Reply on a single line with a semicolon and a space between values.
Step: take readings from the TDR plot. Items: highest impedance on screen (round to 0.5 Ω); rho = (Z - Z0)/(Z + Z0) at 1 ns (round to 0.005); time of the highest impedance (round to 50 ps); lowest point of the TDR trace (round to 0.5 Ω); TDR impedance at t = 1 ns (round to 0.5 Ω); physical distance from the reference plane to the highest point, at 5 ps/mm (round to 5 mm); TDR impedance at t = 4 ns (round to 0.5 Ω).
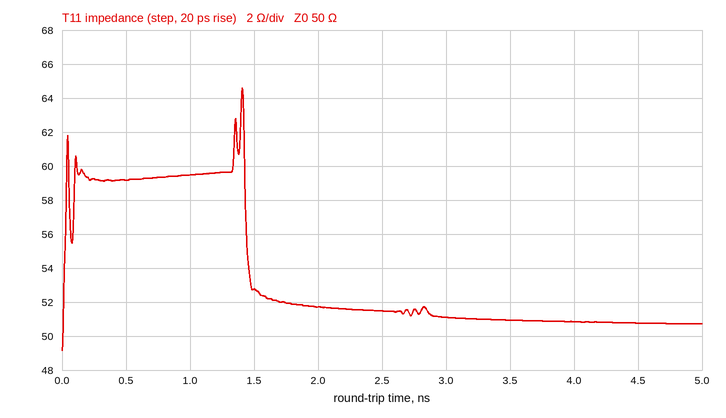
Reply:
64.5 Ω; +0.085; 1.40 ns; 49.0 Ω; 59.5 Ω; 140 mm; 51.0 Ω
